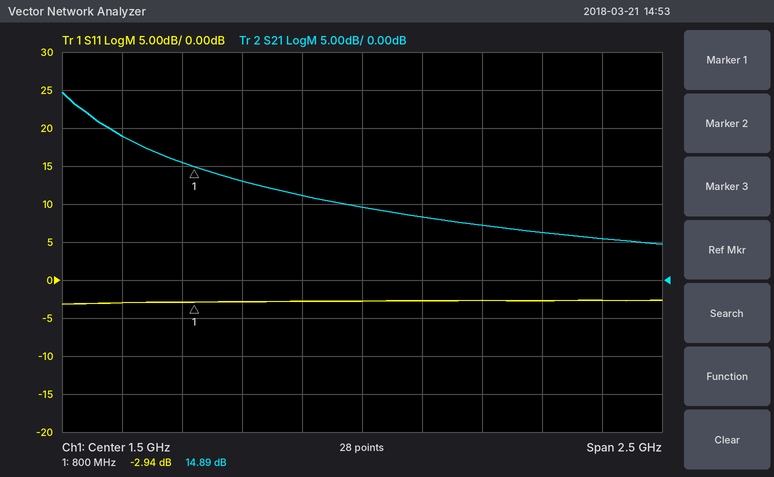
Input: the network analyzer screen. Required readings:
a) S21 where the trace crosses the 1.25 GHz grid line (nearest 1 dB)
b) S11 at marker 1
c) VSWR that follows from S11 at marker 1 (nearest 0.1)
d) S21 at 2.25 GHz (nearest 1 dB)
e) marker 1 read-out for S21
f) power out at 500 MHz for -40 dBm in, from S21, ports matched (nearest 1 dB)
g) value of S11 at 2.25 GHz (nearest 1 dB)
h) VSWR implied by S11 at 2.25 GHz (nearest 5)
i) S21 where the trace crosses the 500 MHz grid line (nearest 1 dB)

11 dB
-2.94 dB
6.0
6 dB
14.89 dB
-21 dBm
-3 dB
5
19 dB
